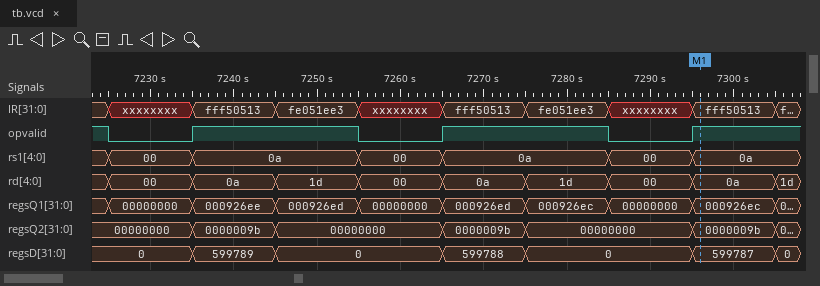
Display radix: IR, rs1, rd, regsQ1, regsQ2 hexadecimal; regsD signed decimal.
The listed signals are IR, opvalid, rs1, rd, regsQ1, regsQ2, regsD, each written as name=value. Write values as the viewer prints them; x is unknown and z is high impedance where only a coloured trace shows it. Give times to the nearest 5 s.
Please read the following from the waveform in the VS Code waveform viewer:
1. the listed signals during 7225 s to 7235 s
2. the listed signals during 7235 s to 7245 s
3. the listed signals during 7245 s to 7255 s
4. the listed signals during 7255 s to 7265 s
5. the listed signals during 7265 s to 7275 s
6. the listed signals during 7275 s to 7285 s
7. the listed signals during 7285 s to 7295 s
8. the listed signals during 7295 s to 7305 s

IR=xxxxxxxx, opvalid=0, rs1=00, rd=00, regsQ1=00000000, regsQ2=00000000, regsD=0
IR=fff50513, opvalid=1, rs1=0a, rd=0a, regsQ1=000926ee, regsQ2=0000009b, regsD=599789
IR=fe051ee3, opvalid=1, rs1=0a, rd=1d, regsQ1=000926ed, regsQ2=00000000, regsD=0
IR=xxxxxxxx, opvalid=0, rs1=00, rd=00, regsQ1=00000000, regsQ2=00000000, regsD=0
IR=fff50513, opvalid=1, rs1=0a, rd=0a, regsQ1=000926ed, regsQ2=0000009b, regsD=599788
IR=fe051ee3, opvalid=1, rs1=0a, rd=1d, regsQ1=000926ec, regsQ2=00000000, regsD=0
IR=xxxxxxxx, opvalid=0, rs1=00, rd=00, regsQ1=00000000, regsQ2=00000000, regsD=0
IR=fff50513, opvalid=1, rs1=0a, rd=0a, regsQ1=000926ec, regsQ2=0000009b, regsD=599787
